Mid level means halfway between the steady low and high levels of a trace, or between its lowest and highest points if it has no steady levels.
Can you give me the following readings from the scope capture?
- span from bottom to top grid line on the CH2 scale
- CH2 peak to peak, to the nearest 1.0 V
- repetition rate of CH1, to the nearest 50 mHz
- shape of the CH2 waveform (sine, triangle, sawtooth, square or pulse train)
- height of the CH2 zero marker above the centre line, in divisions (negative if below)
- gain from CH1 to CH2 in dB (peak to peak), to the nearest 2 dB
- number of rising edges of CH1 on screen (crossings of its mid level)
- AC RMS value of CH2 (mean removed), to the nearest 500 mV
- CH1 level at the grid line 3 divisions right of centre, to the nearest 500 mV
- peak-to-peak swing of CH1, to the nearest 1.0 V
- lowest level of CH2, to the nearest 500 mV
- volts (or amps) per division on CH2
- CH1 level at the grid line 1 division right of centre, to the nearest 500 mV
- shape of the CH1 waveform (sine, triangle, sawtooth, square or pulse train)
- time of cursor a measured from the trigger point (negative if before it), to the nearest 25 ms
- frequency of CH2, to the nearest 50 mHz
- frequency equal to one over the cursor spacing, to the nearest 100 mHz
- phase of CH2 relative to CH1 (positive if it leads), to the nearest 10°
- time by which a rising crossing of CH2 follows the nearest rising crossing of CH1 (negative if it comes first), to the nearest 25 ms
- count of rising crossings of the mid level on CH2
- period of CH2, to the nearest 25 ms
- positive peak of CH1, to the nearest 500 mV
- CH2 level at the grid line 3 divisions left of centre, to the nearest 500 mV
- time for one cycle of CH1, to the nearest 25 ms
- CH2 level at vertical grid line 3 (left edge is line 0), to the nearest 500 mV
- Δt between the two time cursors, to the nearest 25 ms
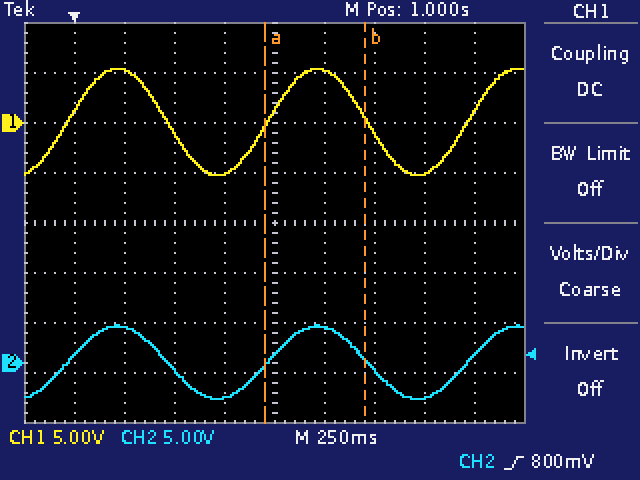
40 V
7.0 V
1.00 Hz
sine
-2.8 div
-4 dB
3
2.5 V
-5.0 V
11.0 V
-3.5 V
5 V
5.5 V
sine
+950 ms
1.00 Hz
2.0 Hz
0°
0 ms
3
1.000 s
5.5 V
3.5 V
1.000 s
-500 mV
500 ms
